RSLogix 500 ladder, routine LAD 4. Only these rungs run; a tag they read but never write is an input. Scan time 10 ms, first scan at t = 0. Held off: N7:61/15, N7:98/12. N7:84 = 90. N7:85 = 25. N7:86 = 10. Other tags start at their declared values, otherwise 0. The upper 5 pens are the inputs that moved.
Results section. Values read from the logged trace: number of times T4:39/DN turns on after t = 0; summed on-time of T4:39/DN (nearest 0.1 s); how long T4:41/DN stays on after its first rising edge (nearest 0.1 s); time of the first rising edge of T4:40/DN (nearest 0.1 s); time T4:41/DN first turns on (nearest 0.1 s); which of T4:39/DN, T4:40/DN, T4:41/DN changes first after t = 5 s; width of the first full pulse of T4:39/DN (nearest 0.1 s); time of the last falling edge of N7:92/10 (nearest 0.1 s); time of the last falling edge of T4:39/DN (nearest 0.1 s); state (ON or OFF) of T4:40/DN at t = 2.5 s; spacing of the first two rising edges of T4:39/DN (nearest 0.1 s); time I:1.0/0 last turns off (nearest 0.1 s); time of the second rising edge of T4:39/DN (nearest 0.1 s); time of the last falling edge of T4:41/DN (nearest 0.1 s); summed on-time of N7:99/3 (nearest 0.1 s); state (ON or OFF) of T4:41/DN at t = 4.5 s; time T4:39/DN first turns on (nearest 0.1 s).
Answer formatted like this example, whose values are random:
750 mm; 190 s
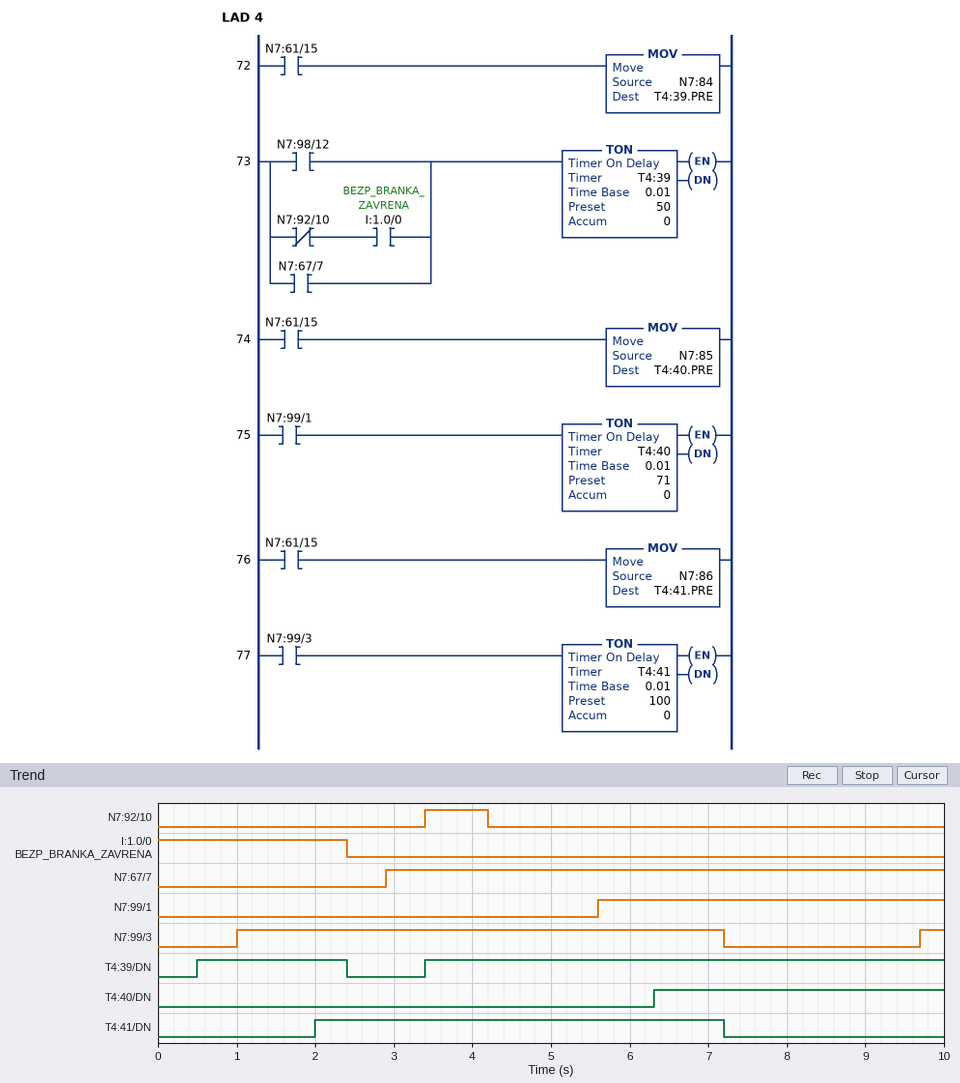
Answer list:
2; 8.5 s; 5.2 s; 6.3 s; 2.0 s; T4:40/DN; 1.9 s; 4.2 s; 2.4 s; OFF; 2.9 s; 2.4 s; 3.4 s; 7.2 s; 6.5 s; ON; 0.5 s
